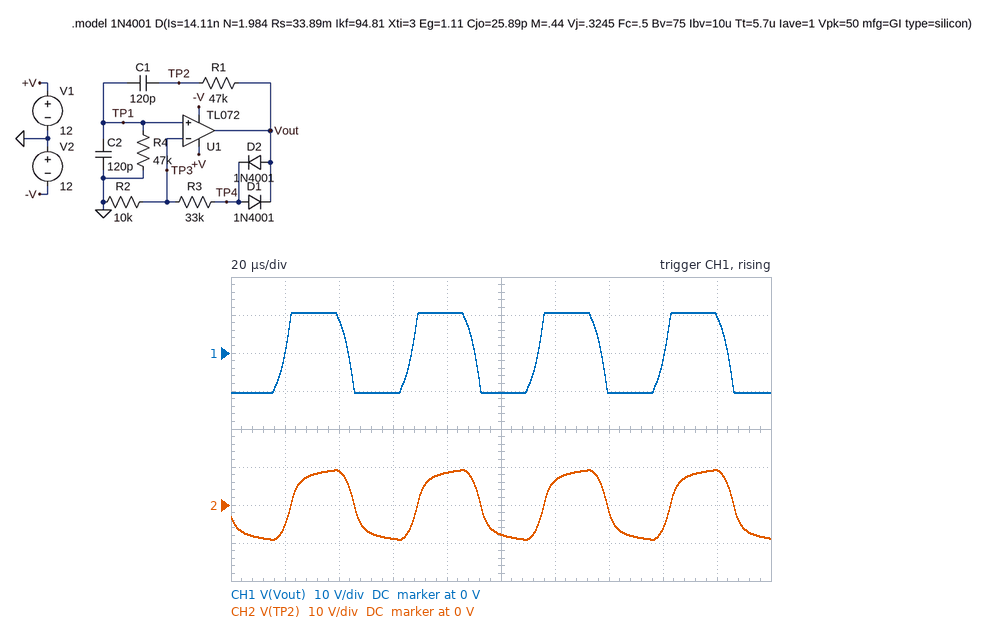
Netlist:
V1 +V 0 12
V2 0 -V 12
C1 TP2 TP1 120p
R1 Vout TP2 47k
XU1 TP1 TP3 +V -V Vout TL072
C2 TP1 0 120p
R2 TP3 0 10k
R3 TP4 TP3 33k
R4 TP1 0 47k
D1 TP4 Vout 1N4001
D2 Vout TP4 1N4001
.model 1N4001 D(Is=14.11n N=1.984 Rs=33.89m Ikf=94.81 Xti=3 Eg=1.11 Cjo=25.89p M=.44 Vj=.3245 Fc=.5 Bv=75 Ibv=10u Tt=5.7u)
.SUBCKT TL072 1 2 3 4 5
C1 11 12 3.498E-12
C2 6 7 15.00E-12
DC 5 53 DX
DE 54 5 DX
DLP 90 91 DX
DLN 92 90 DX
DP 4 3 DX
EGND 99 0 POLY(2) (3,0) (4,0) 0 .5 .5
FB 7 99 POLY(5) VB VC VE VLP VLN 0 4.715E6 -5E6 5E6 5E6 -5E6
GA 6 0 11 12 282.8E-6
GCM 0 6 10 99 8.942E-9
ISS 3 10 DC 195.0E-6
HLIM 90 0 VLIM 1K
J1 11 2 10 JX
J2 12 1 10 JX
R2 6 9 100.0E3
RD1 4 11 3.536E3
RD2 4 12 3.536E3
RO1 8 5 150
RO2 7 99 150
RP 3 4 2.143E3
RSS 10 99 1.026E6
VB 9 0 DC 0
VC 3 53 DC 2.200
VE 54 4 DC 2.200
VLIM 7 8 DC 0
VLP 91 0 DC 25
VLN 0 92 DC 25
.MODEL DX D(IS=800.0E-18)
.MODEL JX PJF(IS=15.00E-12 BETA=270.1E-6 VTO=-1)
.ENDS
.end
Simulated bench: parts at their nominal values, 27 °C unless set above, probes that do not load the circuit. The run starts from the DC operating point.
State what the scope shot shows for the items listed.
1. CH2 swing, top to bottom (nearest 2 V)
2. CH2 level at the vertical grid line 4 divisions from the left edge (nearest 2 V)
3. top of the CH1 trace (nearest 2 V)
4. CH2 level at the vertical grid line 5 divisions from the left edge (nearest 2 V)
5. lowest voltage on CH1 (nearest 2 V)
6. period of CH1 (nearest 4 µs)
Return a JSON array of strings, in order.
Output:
["18 V", "8 V", "10 V", "-8 V", "-10 V", "48 µs"]
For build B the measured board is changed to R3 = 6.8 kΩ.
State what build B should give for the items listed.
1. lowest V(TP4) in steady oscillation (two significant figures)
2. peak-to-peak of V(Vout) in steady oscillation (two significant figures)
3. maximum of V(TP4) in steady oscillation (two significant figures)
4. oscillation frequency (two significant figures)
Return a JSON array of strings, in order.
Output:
["-520 mV", "1.8 V", "520 mV", "16 kHz"]
